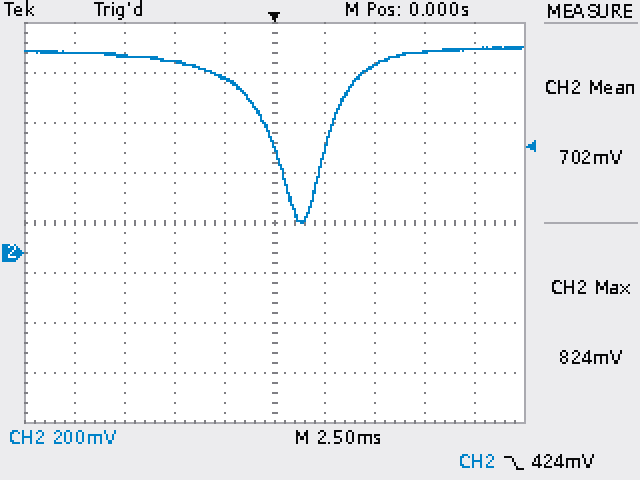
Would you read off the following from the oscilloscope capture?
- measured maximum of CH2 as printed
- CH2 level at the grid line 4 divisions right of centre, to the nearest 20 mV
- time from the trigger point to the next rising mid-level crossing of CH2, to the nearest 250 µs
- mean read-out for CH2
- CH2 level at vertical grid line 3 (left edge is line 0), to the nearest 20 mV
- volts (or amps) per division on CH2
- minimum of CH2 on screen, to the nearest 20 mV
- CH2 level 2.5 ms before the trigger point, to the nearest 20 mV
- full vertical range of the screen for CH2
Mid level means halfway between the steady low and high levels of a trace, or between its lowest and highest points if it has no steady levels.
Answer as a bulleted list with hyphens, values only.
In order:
- 824 mV
- 820 mV
- 2.75 ms
- 702 mV
- 760 mV
- 200 mV
- 120 mV
- 700 mV
- 1.6 V
